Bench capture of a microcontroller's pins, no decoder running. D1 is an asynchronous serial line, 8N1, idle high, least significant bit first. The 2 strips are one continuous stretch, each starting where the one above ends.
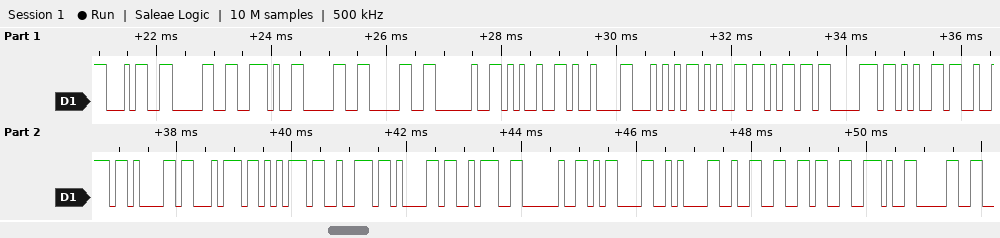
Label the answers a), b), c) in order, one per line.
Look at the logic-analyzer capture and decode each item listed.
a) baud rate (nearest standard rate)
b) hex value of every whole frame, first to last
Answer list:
a) 9600 baud
b) 34 30 2E 30 30 20 25 09 54 65 6D 70 65 72 61 74 75 72 61 3A 20 0D 0A 32 36 2E 30
